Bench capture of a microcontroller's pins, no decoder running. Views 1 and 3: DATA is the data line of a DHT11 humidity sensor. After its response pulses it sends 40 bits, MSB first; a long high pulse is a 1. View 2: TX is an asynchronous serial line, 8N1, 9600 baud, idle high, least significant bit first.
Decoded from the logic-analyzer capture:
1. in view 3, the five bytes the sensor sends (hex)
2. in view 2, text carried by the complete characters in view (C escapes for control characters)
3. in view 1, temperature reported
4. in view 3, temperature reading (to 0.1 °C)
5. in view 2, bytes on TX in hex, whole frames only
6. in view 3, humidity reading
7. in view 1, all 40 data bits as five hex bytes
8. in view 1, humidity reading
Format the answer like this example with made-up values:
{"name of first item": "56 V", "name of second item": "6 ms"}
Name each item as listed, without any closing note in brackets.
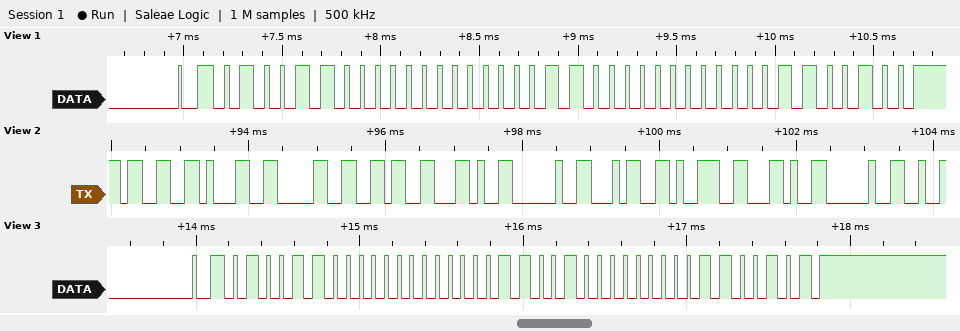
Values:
{"in view 3, the five bytes the sensor sends": "4C 00 19 00 65", "in view 2, text carried by the complete characters in view": "\"3106, 49, \"", "in view 1, temperature reported": "24.0 °C", "in view 3, temperature reading": "25.0 °C", "in view 2, bytes on TX in hex, whole frames only": "33 31 30 36 2C 20 34 39 2C 20", "in view 3, humidity reading": "76 %", "in view 1, all 40 data bits as five hex bytes": "4C 00 18 00 64", "in view 1, humidity reading": "76 %"}
